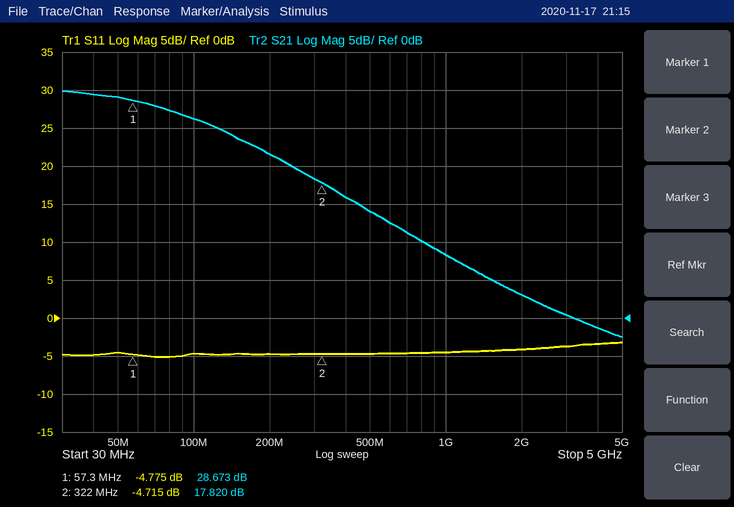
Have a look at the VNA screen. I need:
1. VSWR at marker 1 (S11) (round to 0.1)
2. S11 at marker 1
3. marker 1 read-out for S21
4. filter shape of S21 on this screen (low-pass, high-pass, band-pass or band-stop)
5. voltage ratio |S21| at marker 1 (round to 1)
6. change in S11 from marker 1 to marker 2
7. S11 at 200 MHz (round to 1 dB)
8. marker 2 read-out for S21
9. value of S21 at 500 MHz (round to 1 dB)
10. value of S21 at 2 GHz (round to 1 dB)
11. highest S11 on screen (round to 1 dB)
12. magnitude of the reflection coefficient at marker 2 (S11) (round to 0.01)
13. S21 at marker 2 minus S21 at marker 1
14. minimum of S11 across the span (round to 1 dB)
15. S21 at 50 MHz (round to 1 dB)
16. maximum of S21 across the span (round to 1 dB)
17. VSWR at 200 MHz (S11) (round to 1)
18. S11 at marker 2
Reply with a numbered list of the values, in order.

1. 3.7
2. -4.775 dB
3. 28.673 dB
4. low-pass
5. 27
6. 0.060 dB
7. -5 dB
8. 17.820 dB
9. 14 dB
10. 3 dB
11. -3 dB
12. 0.58
13. -10.853 dB
14. -5 dB
15. 29 dB
16. 30 dB
17. 4
18. -4.715 dB
